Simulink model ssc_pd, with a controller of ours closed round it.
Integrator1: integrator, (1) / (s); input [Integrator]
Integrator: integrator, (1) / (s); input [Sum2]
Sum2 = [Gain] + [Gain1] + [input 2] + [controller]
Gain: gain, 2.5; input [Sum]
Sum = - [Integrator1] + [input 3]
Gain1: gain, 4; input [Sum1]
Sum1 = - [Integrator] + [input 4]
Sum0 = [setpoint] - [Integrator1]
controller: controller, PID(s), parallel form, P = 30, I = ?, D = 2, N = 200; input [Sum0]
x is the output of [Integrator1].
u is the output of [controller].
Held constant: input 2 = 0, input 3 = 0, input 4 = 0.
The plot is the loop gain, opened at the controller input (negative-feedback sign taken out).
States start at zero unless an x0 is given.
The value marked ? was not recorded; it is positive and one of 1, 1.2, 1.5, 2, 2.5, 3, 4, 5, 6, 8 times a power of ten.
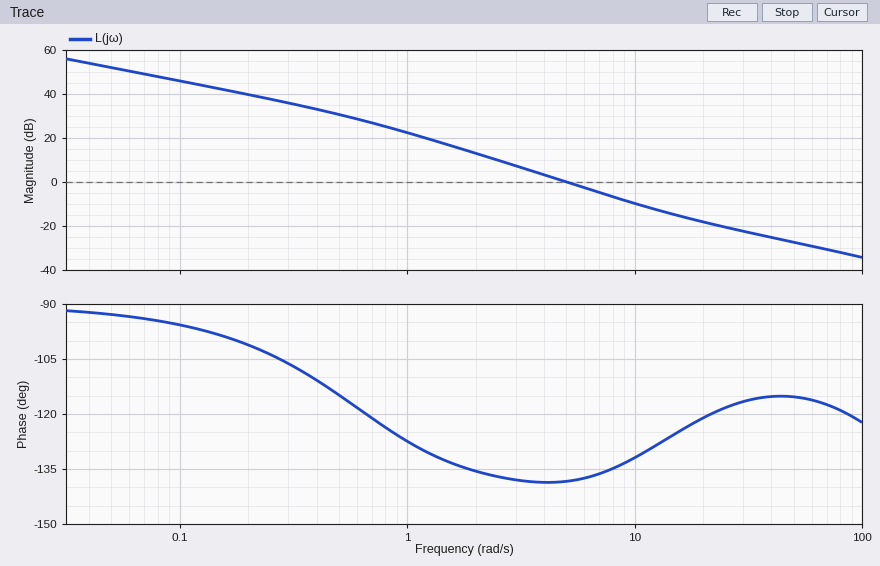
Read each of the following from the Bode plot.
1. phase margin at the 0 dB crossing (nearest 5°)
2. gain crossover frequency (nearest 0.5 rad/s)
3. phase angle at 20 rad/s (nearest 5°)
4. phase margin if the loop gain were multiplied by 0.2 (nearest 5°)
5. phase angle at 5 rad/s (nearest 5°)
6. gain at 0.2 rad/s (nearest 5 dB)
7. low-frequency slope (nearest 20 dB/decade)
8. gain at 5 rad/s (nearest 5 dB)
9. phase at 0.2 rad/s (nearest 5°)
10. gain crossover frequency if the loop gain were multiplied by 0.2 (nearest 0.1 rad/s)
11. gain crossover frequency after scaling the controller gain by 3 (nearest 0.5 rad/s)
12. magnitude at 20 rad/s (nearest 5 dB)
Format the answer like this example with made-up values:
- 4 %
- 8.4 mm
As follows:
- 40°
- 5.0 rad/s
- -120°
- 45°
- -140°
- 40 dB
- -20 dB/decade
- 0 dB
- -100°
- 1.9 rad/s
- 10.0 rad/s
- -20 dB
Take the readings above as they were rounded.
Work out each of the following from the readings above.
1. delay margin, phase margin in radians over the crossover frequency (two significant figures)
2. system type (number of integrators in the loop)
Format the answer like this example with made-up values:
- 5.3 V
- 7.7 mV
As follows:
- 0.14 s
- 1
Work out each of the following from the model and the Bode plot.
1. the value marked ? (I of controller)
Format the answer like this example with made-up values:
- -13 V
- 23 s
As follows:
- 50
